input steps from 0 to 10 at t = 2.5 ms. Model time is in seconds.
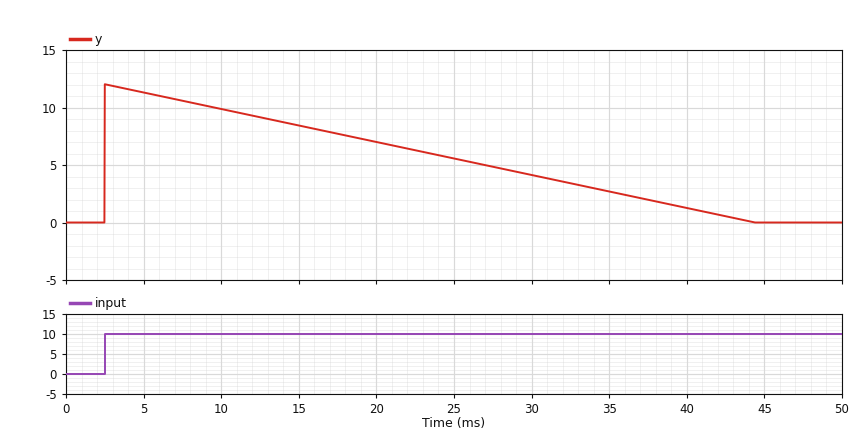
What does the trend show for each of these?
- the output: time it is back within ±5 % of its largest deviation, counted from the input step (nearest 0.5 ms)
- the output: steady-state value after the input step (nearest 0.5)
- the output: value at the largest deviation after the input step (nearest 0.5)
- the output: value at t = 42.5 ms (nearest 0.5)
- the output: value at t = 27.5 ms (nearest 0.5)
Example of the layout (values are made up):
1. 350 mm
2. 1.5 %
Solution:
1. 40.0 ms
2. 0.0
3. 12.0
4. 0.5
5. 5.0
